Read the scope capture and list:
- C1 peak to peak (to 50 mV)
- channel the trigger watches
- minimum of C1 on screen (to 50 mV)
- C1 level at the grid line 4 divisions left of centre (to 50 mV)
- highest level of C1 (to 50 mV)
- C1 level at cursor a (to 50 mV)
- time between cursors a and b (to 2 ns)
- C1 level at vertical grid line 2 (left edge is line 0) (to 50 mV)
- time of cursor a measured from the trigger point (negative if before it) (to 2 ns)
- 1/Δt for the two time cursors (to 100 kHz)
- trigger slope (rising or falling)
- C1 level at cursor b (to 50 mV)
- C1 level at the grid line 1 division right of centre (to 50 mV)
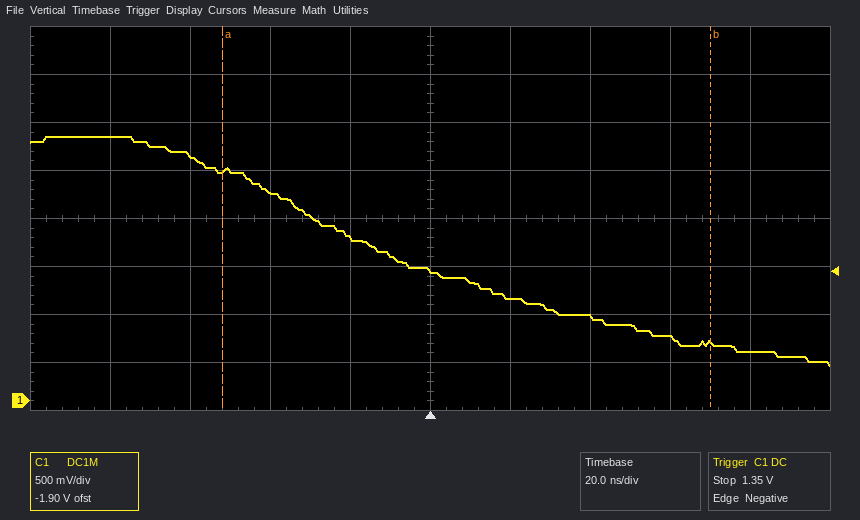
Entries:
2.40 V
C1
350 mV
2.75 V
2.75 V
2.40 V
122 ns
2.55 V
-52 ns
8.2 MHz
falling
600 mV
1.05 V
